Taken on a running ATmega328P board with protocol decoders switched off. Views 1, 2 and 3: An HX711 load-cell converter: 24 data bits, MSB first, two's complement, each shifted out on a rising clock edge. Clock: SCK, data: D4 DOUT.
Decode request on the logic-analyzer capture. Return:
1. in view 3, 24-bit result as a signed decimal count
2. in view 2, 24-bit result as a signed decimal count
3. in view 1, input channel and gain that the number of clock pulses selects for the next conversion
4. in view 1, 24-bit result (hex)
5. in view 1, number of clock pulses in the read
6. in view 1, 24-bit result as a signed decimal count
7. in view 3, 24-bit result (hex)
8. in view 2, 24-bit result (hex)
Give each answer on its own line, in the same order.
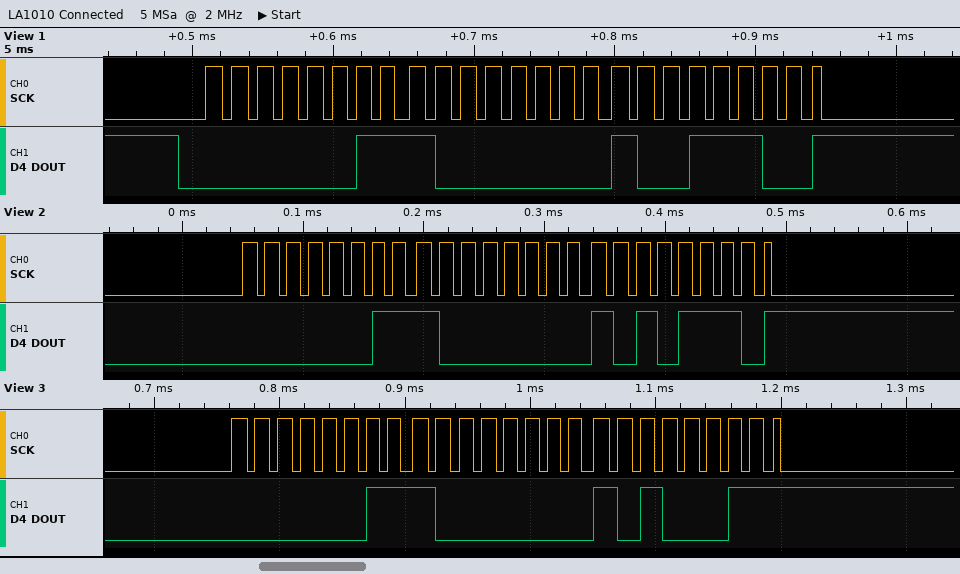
229539
229550
channel A, gain 128
0x03809C
25
229532
0x0380A3
0x0380AE
